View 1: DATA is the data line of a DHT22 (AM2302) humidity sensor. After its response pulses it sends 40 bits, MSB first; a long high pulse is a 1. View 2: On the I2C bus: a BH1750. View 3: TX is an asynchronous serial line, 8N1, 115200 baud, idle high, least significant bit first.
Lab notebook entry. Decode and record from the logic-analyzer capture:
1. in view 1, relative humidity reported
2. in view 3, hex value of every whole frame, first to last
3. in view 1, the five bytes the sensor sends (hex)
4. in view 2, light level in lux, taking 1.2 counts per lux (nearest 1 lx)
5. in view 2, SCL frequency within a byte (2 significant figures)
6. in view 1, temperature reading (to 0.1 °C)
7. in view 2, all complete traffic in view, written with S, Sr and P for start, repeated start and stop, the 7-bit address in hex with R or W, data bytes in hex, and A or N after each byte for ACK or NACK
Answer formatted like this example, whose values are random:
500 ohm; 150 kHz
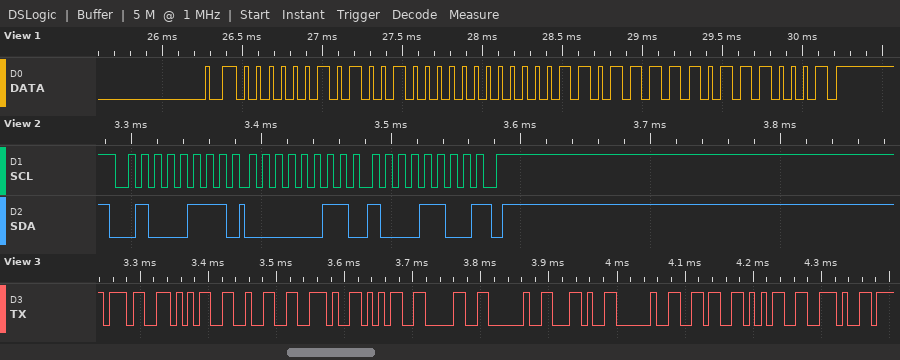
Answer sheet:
65.6 %; 37 35 32 2E 35 30 20 2C 20 36 35 2E; 02 90 00 DF 71; 757 lx; 100 kHz; 22.3 °C; S 23R A 03 A 8C N P
